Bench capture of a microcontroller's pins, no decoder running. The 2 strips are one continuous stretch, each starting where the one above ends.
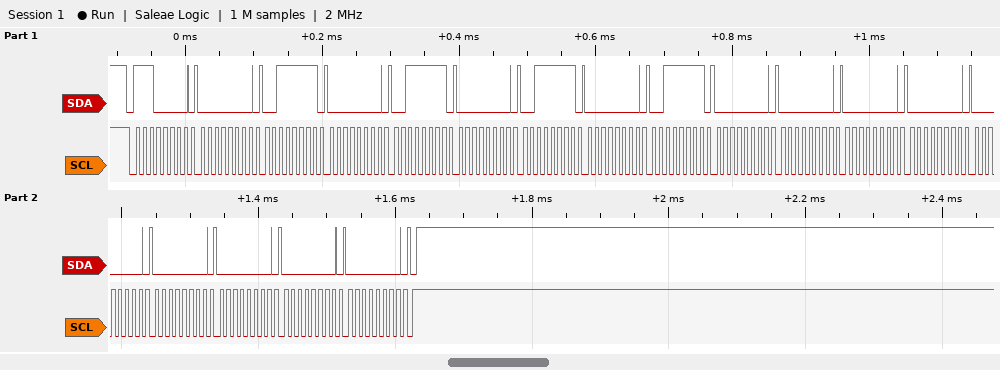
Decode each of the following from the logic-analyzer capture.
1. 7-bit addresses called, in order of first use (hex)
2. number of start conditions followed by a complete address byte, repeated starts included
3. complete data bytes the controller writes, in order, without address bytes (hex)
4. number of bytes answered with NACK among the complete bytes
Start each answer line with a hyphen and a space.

- 0x70
- 1
- 00 3F 00 3F 00 3F 00 3F 00 00 00 00 00 00 00 00 00
- 0
